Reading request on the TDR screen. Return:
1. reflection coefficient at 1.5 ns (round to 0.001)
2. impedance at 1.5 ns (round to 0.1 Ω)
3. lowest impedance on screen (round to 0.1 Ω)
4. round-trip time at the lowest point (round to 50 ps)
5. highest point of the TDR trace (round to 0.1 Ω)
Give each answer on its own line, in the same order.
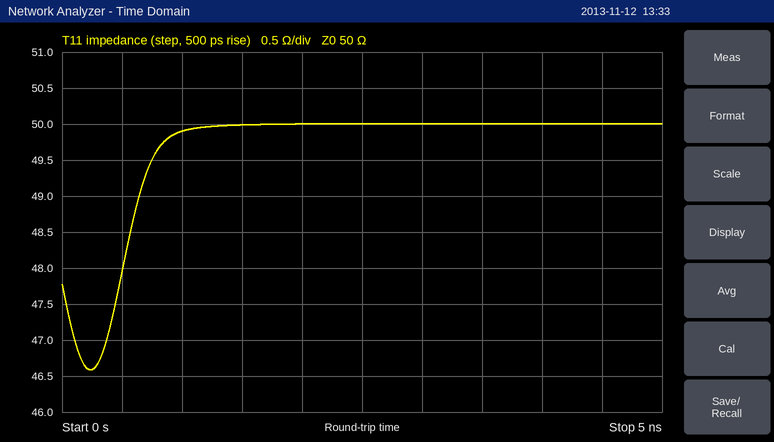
0.000
50.0 Ω
46.6 Ω
250 ps
50.0 Ω
